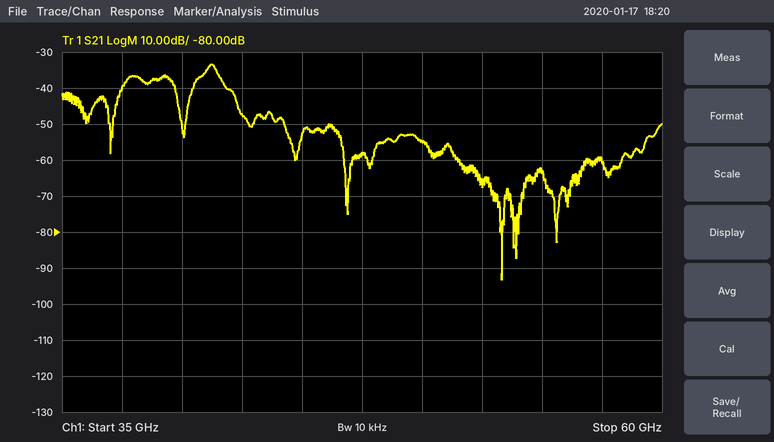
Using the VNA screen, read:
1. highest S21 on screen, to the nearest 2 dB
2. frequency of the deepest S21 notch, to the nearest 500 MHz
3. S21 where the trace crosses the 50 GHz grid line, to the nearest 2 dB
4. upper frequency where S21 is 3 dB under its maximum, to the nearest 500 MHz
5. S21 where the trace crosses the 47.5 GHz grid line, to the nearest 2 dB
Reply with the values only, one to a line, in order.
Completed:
-34 dB
53.5 GHz
-54 dB
41.5 GHz
-58 dB
